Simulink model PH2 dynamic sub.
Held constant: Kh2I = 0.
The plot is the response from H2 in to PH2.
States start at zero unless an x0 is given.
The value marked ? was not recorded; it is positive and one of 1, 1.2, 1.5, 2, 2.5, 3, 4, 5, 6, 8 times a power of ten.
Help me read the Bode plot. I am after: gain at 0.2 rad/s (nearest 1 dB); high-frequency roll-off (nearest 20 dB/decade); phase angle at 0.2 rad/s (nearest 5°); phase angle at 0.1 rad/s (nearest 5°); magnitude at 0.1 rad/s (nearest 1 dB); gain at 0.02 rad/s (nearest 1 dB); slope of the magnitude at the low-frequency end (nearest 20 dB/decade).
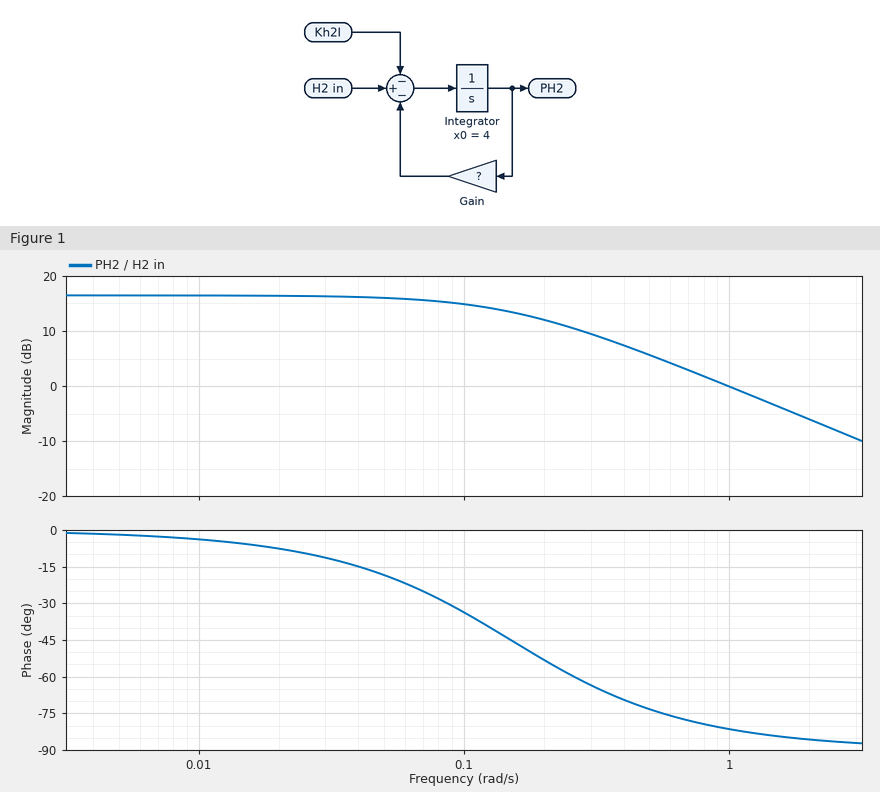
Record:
12 dB
-20 dB/decade
-55°
-35°
15 dB
16 dB
0 dB/decade
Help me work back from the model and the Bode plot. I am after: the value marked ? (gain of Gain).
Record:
0.15
